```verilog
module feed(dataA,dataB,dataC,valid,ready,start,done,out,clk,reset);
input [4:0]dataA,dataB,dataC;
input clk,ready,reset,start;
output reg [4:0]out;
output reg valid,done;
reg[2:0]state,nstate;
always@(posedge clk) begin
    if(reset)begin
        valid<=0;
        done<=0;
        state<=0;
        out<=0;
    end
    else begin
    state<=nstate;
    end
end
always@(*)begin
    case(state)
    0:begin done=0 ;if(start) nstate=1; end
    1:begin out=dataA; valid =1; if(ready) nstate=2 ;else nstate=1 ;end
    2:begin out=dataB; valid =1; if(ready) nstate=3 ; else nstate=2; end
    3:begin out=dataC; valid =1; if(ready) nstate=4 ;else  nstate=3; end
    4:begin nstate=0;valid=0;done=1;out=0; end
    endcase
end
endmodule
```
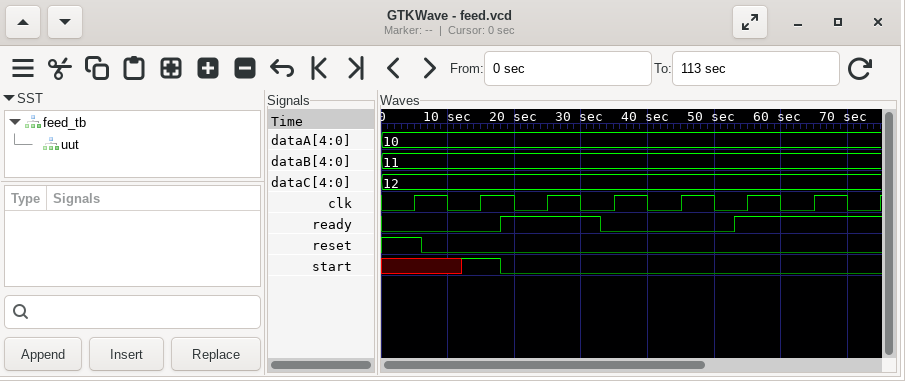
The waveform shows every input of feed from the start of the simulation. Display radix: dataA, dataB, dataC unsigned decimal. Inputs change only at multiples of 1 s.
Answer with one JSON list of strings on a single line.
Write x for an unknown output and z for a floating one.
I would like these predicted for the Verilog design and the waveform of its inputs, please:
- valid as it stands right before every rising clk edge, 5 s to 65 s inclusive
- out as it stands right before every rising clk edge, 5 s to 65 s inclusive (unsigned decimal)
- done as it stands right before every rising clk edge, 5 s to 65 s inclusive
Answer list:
["x 0 1 1 1 1 1", "x, 0, 10, 11, 11, 11, 12", "x 0 0 0 0 0 0"]
